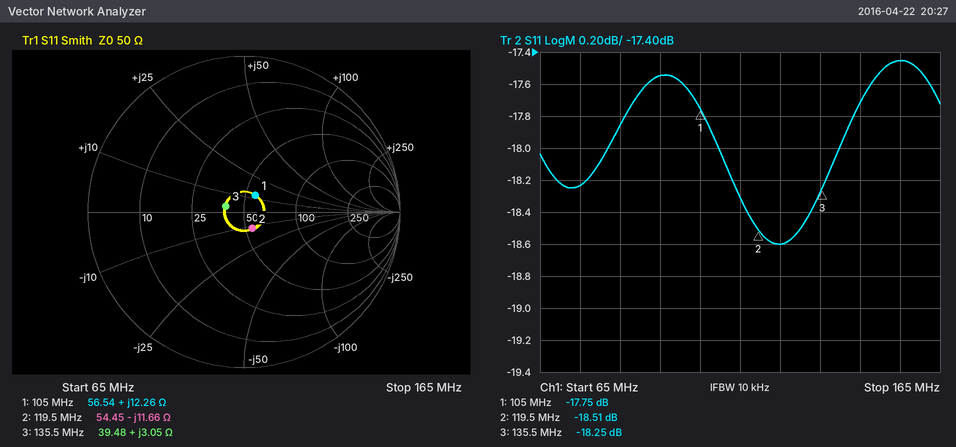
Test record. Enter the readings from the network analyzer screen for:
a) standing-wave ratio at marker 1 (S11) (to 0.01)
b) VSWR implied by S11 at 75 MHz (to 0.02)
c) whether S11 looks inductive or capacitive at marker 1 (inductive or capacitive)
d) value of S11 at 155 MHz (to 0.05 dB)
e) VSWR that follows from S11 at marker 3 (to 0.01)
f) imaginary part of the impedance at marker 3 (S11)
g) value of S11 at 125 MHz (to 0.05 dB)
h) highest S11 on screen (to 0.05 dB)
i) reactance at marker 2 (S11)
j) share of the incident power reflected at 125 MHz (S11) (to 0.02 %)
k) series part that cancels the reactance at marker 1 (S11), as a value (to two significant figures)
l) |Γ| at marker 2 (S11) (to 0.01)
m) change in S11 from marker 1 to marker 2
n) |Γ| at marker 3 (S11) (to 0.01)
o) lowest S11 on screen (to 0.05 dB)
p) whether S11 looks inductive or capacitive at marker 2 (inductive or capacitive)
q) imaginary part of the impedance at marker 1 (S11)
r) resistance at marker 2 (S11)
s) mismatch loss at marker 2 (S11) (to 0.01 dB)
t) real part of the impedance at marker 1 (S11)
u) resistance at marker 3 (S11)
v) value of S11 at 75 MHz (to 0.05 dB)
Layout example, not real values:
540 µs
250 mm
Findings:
1.30
1.28
inductive
-17.45 dB
1.28
+3.05 Ω
-18.60 dB
-17.45 dB
-11.66 Ω
1.38 %
120 pF
0.12
-0.76 dB
0.12
-18.60 dB
capacitive
+12.26 Ω
54.45 Ω
0.06 dB
56.54 Ω
39.48 Ω
-18.25 dB
